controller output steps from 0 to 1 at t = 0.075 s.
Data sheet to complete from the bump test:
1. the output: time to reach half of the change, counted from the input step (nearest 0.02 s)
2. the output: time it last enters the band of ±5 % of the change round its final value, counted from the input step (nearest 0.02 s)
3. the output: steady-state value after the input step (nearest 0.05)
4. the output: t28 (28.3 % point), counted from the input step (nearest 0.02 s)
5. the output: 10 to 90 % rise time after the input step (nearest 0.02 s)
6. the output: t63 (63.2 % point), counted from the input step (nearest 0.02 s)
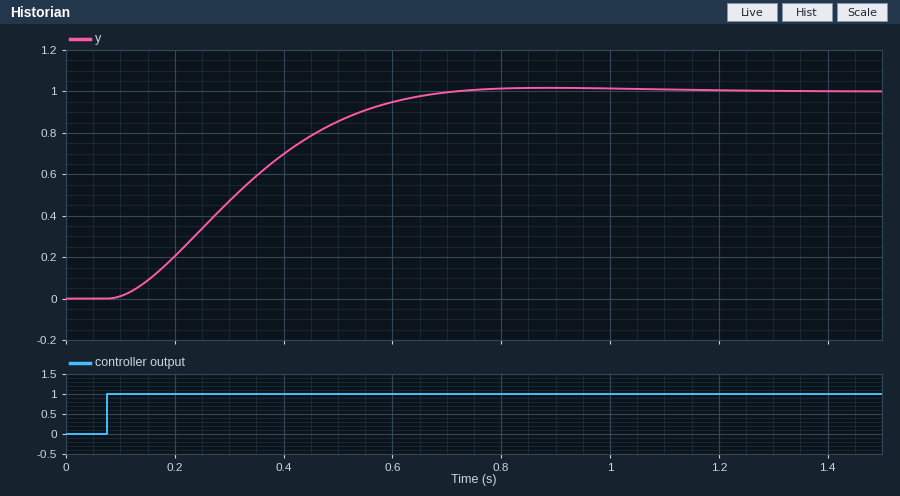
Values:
0.24 s
0.52 s
1.00
0.16 s
0.38 s
0.30 s
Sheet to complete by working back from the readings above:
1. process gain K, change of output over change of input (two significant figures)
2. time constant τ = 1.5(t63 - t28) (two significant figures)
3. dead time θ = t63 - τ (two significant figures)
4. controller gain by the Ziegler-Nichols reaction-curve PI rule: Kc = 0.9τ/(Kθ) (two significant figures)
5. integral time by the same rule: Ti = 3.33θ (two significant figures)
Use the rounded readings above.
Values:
1.0
0.21 s
0.090 s
2.1
0.30 s
